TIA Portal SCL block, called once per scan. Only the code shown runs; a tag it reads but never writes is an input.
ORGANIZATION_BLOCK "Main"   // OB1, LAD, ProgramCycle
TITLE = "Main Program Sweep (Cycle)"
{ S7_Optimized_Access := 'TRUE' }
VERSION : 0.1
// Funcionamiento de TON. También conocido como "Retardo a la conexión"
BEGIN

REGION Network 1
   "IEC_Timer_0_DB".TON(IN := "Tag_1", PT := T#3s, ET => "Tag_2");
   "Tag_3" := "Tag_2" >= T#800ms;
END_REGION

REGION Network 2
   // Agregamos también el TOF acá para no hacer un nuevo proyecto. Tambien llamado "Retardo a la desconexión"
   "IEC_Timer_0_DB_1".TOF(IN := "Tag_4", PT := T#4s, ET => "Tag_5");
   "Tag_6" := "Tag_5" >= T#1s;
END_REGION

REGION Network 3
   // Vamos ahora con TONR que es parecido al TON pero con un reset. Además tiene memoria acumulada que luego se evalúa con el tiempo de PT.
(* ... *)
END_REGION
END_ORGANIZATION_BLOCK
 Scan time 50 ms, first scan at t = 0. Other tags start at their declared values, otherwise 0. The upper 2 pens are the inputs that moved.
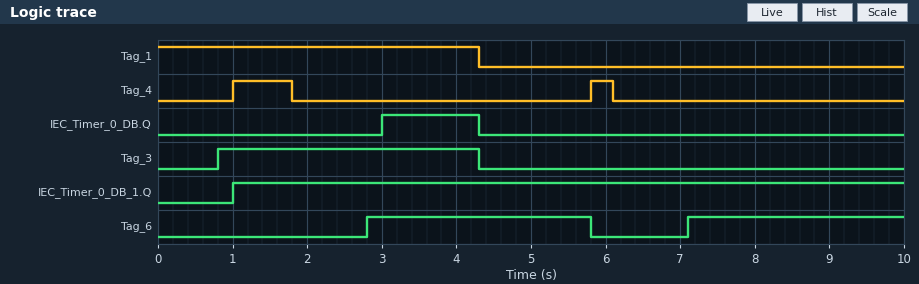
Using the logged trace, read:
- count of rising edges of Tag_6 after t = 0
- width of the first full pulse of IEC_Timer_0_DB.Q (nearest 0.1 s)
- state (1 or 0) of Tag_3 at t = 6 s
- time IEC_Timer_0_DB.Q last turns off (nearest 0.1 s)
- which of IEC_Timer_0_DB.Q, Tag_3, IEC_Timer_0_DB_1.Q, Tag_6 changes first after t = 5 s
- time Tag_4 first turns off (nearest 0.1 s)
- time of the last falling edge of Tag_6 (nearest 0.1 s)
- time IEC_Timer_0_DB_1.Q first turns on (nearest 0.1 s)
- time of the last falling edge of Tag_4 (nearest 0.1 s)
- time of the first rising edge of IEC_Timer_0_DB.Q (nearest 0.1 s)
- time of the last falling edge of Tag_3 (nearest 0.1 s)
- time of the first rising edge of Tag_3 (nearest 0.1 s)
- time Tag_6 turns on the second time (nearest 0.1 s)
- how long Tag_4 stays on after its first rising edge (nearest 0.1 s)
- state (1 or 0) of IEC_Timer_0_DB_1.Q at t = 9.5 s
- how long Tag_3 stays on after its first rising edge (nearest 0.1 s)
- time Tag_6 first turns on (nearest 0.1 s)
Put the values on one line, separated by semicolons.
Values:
2; 1.3 s; 0; 4.3 s; Tag_6; 1.8 s; 5.8 s; 1.0 s; 6.1 s; 3.0 s; 4.3 s; 0.8 s; 7.1 s; 0.8 s; 1; 3.5 s; 2.8 s
